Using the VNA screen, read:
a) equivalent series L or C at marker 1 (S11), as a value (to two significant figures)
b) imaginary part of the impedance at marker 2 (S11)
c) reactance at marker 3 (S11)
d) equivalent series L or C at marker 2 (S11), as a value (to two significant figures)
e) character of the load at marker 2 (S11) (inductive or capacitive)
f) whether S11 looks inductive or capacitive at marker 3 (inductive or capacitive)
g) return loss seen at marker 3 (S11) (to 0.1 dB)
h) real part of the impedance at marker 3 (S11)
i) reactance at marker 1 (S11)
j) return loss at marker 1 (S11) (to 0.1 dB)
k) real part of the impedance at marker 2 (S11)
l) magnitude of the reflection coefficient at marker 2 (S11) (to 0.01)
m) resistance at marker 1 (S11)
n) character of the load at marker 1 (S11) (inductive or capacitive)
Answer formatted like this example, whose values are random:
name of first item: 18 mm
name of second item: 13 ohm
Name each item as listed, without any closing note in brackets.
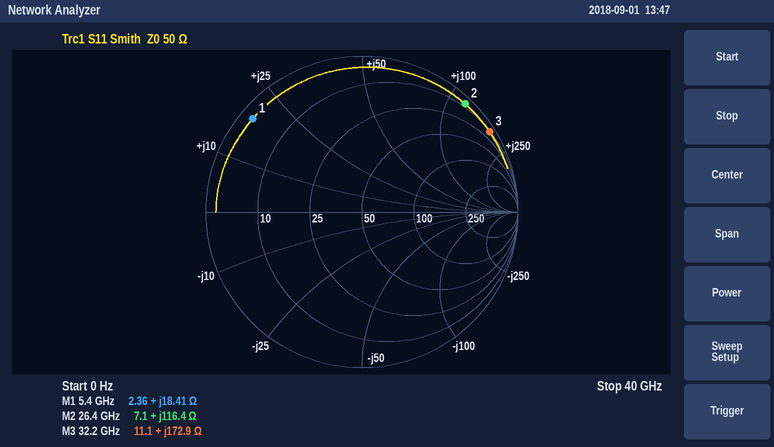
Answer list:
equivalent series L or C at marker 1 (S11), as a value: 540 pH
imaginary part of the impedance at marker 2: +116.4 Ω
reactance at marker 3: +172.9 Ω
equivalent series L or C at marker 2 (S11), as a value: 700 pH
character of the load at marker 2 (S11): inductive
whether S11 looks inductive or capacitive at marker 3: inductive
return loss seen at marker 3 (S11): 0.3 dB
real part of the impedance at marker 3: 11.1 Ω
reactance at marker 1: +18.41 Ω
return loss at marker 1 (S11): 0.7 dB
real part of the impedance at marker 2: 7.1 Ω
magnitude of the reflection coefficient at marker 2 (S11): 0.96
resistance at marker 1: 2.36 Ω
character of the load at marker 1 (S11): inductive
